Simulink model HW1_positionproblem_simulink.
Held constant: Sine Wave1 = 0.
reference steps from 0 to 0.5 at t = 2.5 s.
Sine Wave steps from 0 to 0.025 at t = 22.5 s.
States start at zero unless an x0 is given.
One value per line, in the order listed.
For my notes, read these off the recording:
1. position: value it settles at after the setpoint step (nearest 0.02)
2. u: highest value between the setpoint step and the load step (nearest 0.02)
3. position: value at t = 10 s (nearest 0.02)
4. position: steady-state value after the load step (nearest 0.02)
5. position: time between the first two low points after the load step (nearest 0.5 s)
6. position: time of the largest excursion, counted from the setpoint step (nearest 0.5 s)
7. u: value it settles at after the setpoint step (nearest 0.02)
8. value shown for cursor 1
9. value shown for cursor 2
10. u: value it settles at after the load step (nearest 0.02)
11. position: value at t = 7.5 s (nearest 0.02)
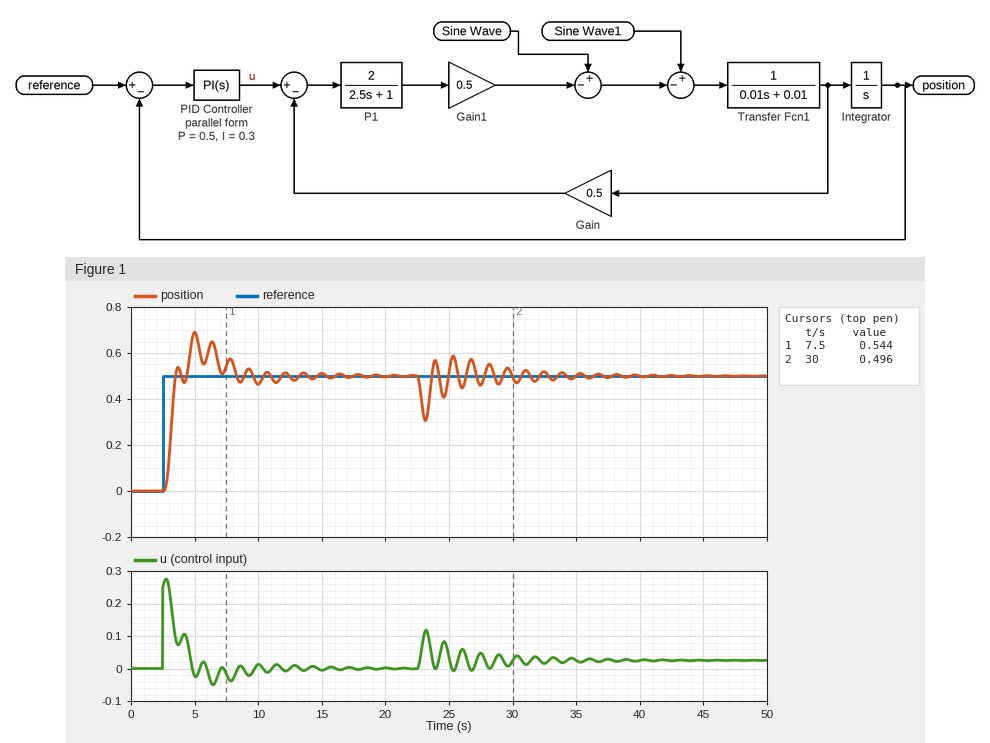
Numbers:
0.50
0.28
0.46
0.50
1.5 s
2.5 s
0.00
0.544
0.496
0.02
0.54
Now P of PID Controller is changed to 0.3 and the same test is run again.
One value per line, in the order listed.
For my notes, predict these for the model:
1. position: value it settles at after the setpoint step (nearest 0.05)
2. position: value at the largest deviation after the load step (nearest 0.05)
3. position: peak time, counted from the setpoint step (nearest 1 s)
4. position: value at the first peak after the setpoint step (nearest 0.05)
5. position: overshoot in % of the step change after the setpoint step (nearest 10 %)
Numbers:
0.50
0.30
3 s
0.70
40 %
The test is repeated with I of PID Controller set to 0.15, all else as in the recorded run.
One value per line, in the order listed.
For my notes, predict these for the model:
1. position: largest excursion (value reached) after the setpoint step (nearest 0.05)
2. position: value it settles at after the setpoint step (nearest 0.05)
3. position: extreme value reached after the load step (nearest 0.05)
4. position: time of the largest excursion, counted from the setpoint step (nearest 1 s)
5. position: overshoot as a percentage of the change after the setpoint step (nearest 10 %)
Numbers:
0.65
0.50
0.30
4 s
30 %
